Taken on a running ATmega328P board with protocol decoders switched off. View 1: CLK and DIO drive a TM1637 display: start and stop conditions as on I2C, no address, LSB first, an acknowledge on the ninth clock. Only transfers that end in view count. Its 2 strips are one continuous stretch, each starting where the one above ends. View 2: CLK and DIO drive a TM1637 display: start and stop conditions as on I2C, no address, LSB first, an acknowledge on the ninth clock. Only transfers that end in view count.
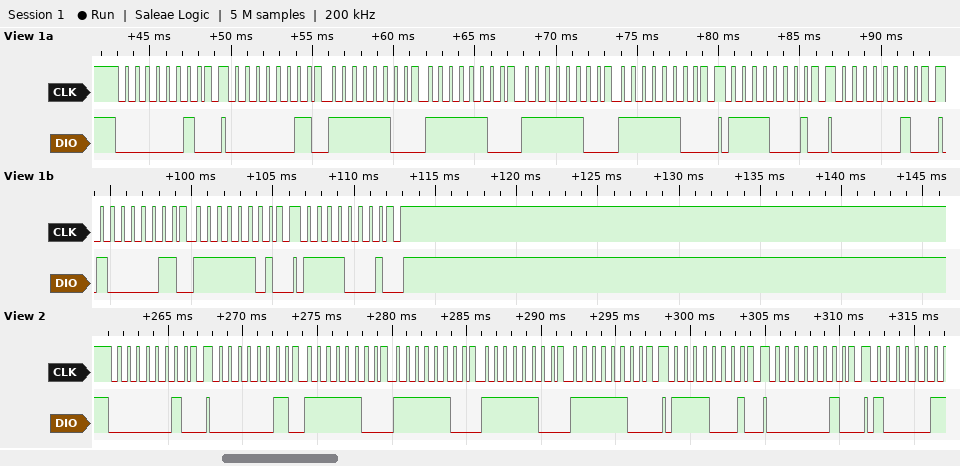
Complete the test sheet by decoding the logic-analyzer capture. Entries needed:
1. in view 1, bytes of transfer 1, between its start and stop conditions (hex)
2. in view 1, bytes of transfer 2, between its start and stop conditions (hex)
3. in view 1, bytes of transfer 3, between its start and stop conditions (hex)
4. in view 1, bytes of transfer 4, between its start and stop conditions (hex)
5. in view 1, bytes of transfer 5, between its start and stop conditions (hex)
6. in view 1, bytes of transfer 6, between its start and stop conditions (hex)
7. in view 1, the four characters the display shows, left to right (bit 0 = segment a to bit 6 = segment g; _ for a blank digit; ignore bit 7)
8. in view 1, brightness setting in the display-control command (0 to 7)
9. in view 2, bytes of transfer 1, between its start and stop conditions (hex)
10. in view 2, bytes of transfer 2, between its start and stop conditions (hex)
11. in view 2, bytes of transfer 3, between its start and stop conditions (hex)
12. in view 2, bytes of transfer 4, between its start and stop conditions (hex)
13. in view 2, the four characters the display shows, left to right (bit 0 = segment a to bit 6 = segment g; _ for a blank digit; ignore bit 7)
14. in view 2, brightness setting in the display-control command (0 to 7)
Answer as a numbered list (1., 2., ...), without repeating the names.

1. 40
2. C0 3F 3F 3F 3F
3. 8F
4. 40
5. C1 BF
6. 8F
7. 0000
8. 7
9. 40
10. C0 3F 3F 3F 3F
11. 8F
12. 40
13. 0000
14. 7
